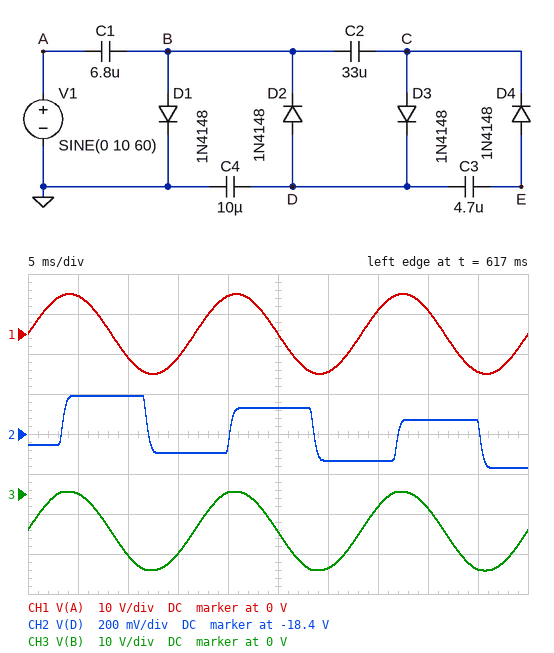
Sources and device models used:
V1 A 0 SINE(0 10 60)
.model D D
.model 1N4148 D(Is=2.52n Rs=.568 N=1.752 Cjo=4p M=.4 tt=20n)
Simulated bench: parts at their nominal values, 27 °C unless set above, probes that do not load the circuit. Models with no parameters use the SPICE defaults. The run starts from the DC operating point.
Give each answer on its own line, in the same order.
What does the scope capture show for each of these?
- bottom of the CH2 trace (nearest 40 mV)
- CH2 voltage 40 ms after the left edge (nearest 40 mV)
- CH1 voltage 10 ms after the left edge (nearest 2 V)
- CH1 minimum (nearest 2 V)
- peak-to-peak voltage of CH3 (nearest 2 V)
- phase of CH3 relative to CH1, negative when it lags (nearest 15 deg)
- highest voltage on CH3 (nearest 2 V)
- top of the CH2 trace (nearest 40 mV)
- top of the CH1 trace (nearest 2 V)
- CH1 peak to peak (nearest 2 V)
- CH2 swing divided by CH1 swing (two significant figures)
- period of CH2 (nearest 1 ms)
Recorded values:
-18.56 V
-18.32 V
-6 V
-10 V
20 V
0 deg
0 V
-18.20 V
10 V
20 V
0.018
17 ms
